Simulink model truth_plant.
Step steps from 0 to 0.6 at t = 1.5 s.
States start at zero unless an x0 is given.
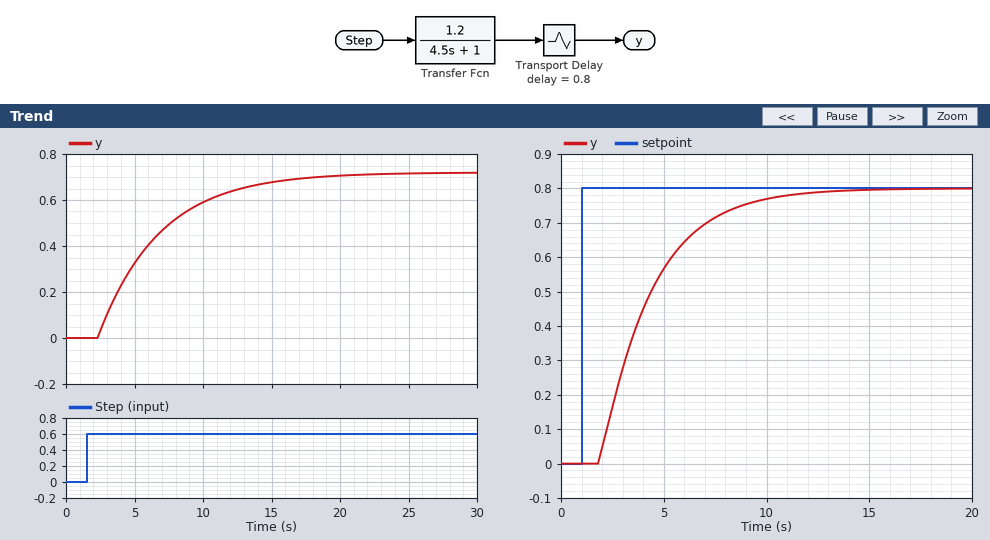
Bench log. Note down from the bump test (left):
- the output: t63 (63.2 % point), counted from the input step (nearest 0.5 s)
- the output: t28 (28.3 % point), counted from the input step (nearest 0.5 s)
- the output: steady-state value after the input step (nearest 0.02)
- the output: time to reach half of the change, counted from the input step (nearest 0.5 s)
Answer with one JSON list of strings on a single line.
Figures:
["5.5 s", "2.5 s", "0.72", "4.0 s"]
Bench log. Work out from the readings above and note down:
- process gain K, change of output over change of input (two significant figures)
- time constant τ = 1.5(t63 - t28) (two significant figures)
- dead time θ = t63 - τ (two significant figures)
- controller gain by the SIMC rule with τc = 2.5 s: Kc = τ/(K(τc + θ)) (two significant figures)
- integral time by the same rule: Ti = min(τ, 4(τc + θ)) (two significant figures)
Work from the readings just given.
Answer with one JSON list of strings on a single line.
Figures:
["1.2", "4.5 s", "1.0 s", "1.1", "4.5 s"]
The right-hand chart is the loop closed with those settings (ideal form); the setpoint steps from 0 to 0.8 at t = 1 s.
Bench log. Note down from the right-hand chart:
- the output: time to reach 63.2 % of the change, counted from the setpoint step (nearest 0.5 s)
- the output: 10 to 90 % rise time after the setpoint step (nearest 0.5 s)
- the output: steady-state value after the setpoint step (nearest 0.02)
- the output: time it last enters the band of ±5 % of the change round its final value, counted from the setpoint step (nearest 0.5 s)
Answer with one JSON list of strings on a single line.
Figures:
["3.5 s", "5.5 s", "0.80", "8.5 s"]
